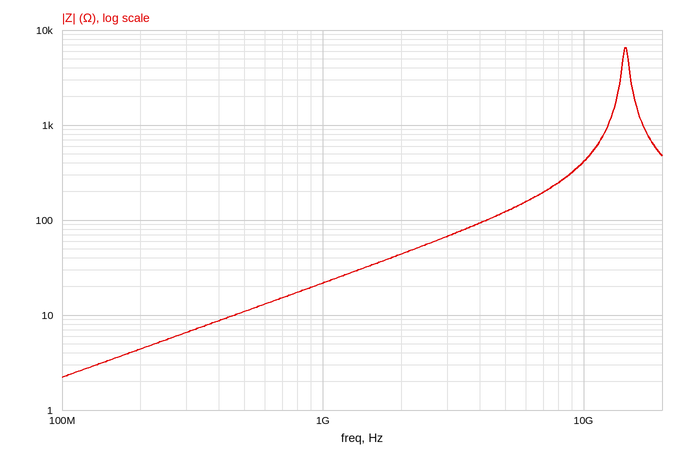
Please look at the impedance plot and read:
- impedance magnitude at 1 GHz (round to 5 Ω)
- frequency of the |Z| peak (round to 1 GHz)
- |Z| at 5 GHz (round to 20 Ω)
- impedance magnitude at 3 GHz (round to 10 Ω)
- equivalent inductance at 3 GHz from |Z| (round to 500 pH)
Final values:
20 Ω
14 GHz
120 Ω
70 Ω
3.5 nH
